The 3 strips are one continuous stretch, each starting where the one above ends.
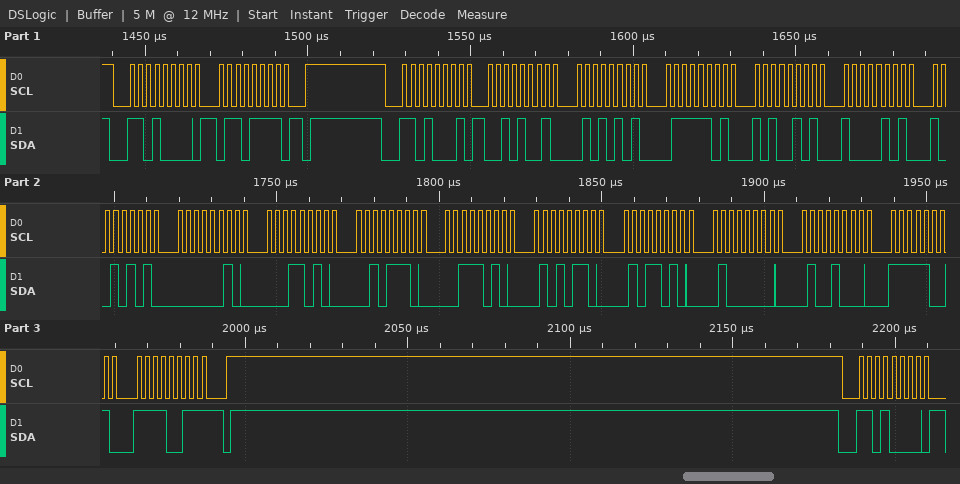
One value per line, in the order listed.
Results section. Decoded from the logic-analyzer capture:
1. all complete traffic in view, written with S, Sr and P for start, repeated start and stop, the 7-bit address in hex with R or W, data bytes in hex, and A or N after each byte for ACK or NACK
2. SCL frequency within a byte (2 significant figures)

S 68W A 6F A P S 68R A 29 A 55 A 7D A A5 A 85 A 95 A 02 A 1A A 2E A 3A A 56 A 5A A 40 A 48 A F9 A F3 N P S 68W A
400 kHz
